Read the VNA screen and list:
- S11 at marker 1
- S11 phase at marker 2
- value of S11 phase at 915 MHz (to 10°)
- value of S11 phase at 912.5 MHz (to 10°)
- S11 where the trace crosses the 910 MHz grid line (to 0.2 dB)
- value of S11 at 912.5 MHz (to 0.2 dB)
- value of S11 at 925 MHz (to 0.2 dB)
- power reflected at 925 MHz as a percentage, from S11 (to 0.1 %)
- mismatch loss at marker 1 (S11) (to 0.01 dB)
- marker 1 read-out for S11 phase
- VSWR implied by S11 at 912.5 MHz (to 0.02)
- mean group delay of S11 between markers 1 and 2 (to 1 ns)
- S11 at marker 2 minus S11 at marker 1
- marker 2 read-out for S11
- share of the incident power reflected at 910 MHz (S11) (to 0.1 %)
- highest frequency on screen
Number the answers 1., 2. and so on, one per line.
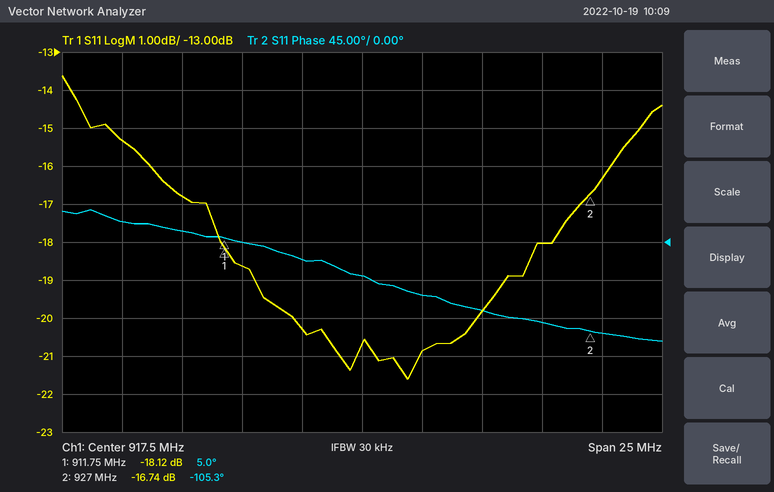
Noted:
1. -18.12 dB
2. -105.3°
3. -20°
4. 0°
5. -16.8 dB
6. -18.6 dB
7. -18.0 dB
8. 1.6 %
9. 0.07 dB
10. 5.0°
11. 1.26
12. 20 ns
13. 1.38 dB
14. -16.74 dB
15. 2.1 %
16. 930 MHz
